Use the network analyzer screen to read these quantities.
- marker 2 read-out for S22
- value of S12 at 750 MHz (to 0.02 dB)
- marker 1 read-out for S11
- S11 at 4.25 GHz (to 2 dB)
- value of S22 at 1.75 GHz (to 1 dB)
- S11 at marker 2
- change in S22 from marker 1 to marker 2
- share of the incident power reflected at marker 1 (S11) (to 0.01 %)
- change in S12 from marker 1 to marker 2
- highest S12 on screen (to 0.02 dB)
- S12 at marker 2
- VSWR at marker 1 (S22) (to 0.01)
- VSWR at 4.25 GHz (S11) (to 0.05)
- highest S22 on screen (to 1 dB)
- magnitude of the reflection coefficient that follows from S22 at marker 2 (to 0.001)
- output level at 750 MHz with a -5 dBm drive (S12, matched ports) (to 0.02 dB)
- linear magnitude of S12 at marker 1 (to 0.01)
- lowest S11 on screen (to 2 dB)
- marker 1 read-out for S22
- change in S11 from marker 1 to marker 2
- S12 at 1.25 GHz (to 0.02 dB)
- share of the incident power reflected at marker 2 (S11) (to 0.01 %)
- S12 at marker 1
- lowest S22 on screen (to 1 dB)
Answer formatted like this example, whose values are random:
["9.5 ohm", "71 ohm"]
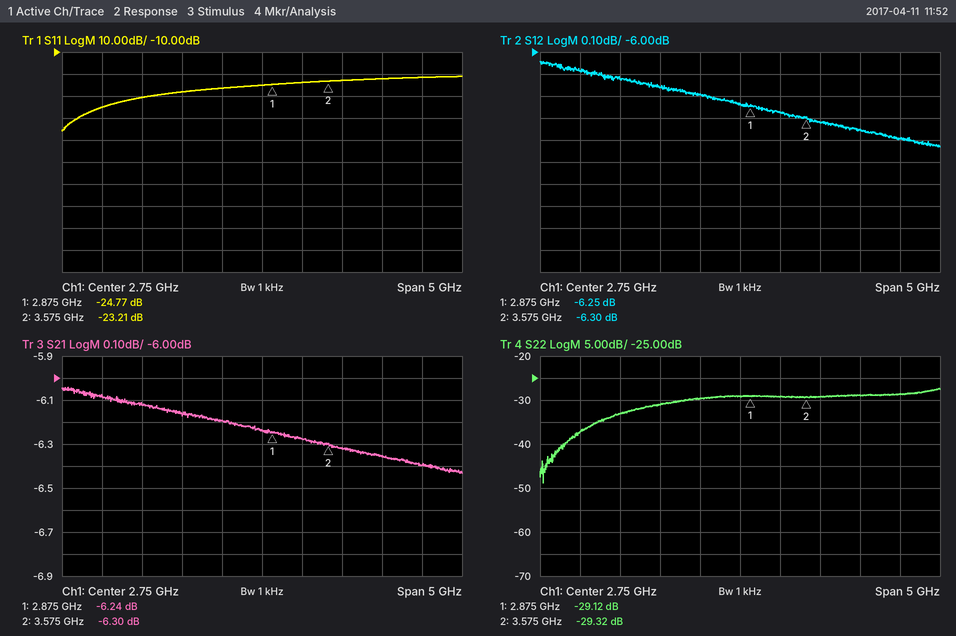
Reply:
["-29.32 dB", "-6.08 dB", "-24.77 dB", "-22 dB", "-31 dB", "-23.21 dB", "-0.20 dB", "0.33 %", "-0.05 dB", "-6.04 dB", "-6.30 dB", "1.07", "1.15", "-27 dB", "0.034", "-11.08 dBm", "0.49", "-46 dB", "-29.12 dB", "1.56 dB", "-6.12 dB", "0.48 %", "-6.25 dB", "-49 dB"]
